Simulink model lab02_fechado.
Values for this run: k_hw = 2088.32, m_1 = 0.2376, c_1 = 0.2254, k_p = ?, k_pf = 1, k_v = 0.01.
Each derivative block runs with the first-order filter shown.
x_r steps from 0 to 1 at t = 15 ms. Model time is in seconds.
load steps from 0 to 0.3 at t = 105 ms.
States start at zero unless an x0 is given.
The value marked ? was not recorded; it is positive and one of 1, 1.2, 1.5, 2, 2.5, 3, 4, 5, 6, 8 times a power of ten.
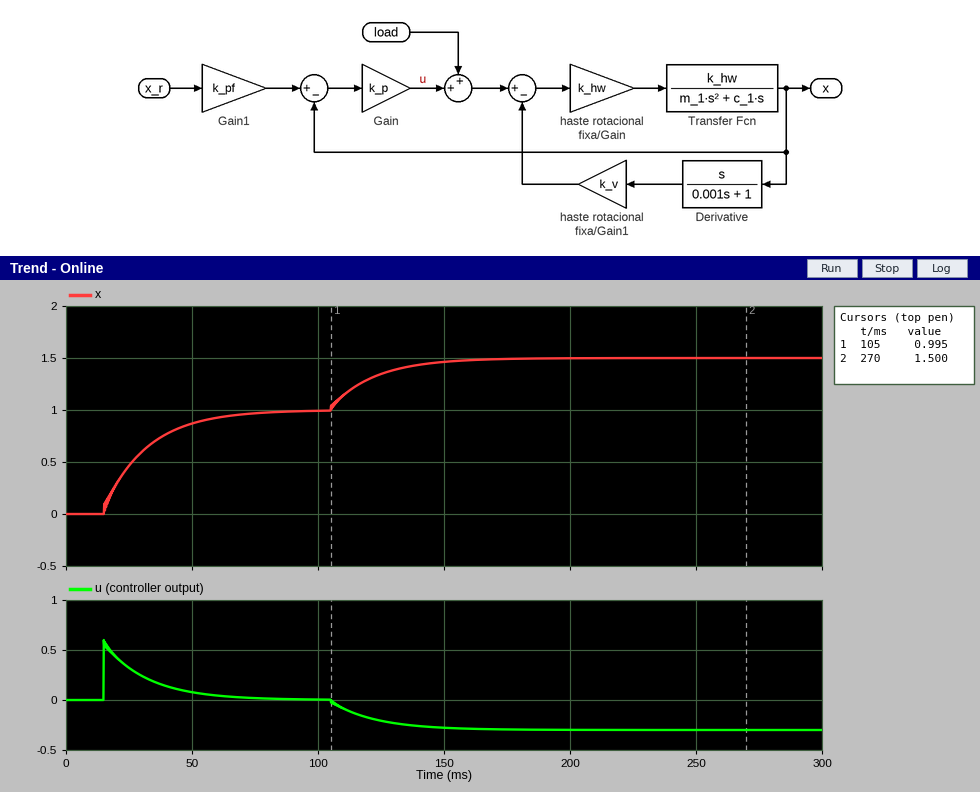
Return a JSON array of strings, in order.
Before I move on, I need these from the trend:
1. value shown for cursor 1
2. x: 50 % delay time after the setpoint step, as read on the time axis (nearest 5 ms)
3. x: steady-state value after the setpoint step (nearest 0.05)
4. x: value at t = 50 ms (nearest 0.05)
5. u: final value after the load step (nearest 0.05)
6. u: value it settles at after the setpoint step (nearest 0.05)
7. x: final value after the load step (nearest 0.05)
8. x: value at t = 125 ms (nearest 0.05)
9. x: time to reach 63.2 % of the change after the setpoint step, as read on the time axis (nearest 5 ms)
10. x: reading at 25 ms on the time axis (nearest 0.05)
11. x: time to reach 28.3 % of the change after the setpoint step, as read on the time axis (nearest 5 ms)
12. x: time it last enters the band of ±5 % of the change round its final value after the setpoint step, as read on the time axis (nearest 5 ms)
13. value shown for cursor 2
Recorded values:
["0.995", "25 ms", "1.00", "0.85", "-0.30", "0.00", "1.50", "1.35", "30 ms", "0.45", "20 ms", "65 ms", "1.500"]
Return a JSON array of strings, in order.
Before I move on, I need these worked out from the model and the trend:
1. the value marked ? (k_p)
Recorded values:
["0.6"]
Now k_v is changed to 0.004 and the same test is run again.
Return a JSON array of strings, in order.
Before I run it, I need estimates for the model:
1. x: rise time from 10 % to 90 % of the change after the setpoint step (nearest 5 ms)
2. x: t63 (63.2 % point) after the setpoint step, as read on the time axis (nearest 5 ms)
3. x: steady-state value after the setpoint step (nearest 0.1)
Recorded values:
["15 ms", "20 ms", "1.0"]
